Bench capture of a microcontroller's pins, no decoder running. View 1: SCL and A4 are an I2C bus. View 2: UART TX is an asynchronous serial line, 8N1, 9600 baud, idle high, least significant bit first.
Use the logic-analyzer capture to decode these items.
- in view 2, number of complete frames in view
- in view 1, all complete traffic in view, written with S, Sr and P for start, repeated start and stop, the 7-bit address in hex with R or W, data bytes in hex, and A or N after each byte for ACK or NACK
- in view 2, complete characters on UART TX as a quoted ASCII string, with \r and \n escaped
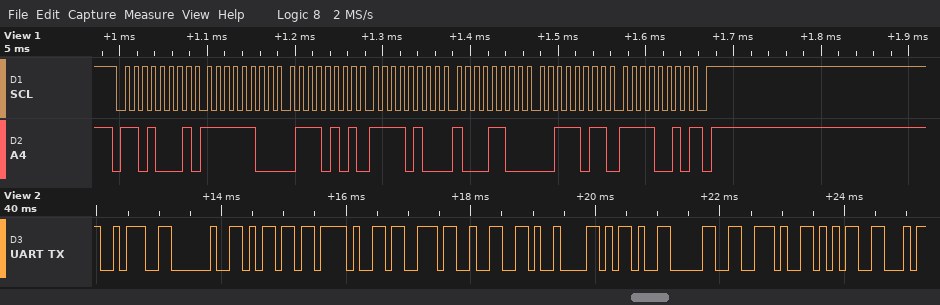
11
S 68R A FC A 75 A F4 A 8C A 3B A F2 N P
": m/s2\t-0.5"
